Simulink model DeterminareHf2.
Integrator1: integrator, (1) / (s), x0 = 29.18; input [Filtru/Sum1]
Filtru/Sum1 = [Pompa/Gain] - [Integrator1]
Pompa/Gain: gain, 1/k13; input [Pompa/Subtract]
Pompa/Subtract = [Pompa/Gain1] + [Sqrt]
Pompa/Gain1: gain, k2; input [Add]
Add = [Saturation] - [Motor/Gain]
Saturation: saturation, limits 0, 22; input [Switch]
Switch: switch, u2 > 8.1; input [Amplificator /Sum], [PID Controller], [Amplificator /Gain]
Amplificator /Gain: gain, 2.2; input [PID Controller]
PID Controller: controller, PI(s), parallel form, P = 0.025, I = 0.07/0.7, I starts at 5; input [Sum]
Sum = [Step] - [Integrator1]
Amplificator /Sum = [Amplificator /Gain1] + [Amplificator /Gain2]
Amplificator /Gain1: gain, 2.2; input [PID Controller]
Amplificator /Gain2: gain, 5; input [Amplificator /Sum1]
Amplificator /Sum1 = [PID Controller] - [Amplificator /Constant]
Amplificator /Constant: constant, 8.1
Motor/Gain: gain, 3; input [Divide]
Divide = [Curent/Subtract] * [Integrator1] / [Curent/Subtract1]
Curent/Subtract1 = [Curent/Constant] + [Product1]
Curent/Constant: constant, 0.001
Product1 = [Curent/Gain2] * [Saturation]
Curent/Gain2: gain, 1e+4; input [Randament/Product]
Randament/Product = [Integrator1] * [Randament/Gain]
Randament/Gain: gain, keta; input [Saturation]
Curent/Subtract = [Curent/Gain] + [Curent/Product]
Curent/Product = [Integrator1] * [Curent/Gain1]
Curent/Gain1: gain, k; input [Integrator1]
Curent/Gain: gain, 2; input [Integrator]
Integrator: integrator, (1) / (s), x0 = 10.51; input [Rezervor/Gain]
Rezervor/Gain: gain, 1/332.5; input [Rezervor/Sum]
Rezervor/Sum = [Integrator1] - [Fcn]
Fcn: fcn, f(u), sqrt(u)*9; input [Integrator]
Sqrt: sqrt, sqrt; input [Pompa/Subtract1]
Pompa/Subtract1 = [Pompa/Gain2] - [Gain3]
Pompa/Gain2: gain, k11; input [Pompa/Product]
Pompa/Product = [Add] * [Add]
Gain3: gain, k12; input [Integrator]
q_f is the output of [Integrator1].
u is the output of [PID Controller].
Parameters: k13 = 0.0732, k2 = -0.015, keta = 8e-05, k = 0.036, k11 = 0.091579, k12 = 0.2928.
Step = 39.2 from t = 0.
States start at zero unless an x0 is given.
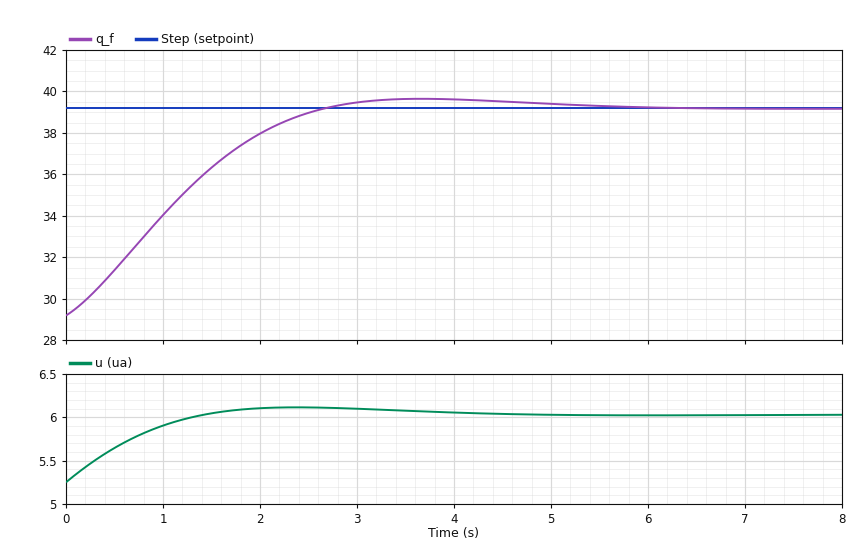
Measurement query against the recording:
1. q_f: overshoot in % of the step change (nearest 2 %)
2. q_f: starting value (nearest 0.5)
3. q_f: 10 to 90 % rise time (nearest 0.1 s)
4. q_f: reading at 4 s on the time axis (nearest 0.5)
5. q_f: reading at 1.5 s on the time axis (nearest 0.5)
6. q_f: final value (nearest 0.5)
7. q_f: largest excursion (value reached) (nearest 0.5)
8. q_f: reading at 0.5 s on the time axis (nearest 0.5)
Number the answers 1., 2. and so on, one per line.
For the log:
1. 4 %
2. 29.0
3. 1.8 s
4. 39.5
5. 36.5
6. 39.0
7. 39.5
8. 31.5
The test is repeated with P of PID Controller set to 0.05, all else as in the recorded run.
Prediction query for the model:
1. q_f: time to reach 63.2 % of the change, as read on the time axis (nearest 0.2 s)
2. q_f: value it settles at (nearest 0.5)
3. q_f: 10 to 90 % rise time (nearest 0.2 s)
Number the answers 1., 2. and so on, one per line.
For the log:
1. 1.2 s
2. 39.0
3. 2.0 s
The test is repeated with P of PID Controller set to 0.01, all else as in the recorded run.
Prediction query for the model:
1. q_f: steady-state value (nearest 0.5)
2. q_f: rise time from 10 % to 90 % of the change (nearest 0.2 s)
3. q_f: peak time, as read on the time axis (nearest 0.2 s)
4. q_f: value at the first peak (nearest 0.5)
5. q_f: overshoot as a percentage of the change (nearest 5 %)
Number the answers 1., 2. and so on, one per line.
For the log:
1. 39.0
2. 1.6 s
3. 3.4 s
4. 40.0
5. 10 %
